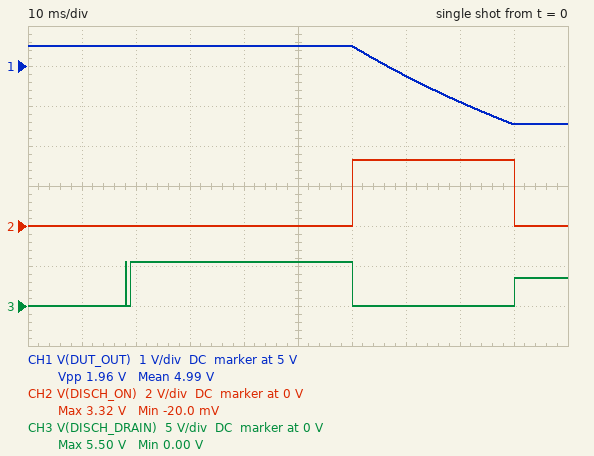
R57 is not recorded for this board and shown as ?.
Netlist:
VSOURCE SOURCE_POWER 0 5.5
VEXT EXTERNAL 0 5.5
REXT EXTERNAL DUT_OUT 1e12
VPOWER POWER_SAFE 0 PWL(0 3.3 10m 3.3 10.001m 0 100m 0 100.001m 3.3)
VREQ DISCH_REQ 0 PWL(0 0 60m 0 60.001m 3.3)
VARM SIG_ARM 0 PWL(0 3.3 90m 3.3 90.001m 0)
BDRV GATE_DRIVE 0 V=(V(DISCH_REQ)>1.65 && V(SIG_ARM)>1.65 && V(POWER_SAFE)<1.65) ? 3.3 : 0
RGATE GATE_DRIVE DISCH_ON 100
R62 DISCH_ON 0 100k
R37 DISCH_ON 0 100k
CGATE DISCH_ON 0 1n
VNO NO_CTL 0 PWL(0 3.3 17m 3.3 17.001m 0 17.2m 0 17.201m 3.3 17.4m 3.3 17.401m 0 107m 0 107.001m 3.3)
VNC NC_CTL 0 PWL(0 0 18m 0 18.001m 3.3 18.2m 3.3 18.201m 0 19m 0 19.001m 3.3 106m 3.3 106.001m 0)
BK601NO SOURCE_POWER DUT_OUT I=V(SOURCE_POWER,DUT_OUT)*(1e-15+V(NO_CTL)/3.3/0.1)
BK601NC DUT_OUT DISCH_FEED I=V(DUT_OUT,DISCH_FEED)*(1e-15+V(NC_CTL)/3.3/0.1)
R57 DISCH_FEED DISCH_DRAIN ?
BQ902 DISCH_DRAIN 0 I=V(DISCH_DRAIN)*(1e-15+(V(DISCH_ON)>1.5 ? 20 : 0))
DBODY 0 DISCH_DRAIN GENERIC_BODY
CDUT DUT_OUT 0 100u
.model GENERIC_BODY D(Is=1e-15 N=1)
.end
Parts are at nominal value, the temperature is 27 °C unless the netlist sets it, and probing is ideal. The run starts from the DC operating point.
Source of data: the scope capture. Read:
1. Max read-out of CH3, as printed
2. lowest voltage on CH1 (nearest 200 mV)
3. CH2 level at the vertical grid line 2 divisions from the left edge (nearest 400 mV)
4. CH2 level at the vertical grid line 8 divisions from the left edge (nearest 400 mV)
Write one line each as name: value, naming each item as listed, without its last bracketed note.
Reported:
Max read-out of CH3, as printed: 5.50 V
lowest voltage on CH1: 3.6 V
CH2 level at the vertical grid line 2 divisions from the left edge: 0 V
CH2 level at the vertical grid line 8 divisions from the left edge: 3.2 V
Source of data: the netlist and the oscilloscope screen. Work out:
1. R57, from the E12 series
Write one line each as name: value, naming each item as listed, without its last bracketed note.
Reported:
R57, from the E12 series: 680 Ω
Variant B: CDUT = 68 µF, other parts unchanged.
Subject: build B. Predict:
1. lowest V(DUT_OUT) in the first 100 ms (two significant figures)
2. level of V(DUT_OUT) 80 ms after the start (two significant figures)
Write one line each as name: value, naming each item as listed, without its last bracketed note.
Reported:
lowest V(DUT_OUT) in the first 100 ms: 2.9 V
level of V(DUT_OUT) 80 ms after the start: 3.6 V
